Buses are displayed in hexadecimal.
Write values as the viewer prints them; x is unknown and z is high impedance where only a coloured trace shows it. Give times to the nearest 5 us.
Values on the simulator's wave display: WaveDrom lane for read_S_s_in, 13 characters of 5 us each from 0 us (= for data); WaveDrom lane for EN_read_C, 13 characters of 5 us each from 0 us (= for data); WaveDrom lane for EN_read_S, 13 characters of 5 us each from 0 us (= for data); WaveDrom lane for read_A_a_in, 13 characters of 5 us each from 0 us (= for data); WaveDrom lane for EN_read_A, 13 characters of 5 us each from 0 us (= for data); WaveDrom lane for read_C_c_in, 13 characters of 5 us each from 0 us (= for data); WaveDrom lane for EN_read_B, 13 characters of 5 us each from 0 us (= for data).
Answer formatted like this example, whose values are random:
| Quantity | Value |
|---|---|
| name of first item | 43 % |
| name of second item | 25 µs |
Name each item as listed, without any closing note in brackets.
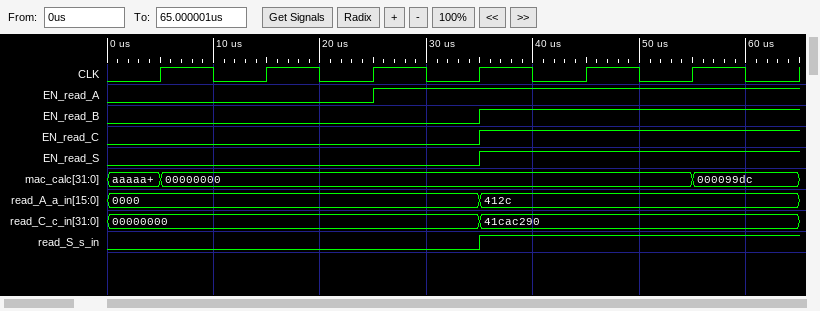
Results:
| Quantity | Value |
|---|---|
| WaveDrom lane for read_S_s_in, 13 characters of 5 us each from 0 us | {name: 'read_S_s_in', wave: '0......1.....'} |
| WaveDrom lane for EN_read_C, 13 characters of 5 us each from 0 us | {name: 'EN_read_C', wave: '0......1.....'} |
| WaveDrom lane for EN_read_S, 13 characters of 5 us each from 0 us | {name: 'EN_read_S', wave: '0......1.....'} |
| WaveDrom lane for read_A_a_in, 13 characters of 5 us each from 0 us | {name: 'read_A_a_in', wave: '=......=.....', data: '0000 412c'} |
| WaveDrom lane for EN_read_A, 13 characters of 5 us each from 0 us | {name: 'EN_read_A', wave: '0....1.......'} |
| WaveDrom lane for read_C_c_in, 13 characters of 5 us each from 0 us | {name: 'read_C_c_in', wave: '=......=.....', data: '00000000 41cac290'} |
| WaveDrom lane for EN_read_B, 13 characters of 5 us each from 0 us | {name: 'EN_read_B', wave: '0......1.....'} |
